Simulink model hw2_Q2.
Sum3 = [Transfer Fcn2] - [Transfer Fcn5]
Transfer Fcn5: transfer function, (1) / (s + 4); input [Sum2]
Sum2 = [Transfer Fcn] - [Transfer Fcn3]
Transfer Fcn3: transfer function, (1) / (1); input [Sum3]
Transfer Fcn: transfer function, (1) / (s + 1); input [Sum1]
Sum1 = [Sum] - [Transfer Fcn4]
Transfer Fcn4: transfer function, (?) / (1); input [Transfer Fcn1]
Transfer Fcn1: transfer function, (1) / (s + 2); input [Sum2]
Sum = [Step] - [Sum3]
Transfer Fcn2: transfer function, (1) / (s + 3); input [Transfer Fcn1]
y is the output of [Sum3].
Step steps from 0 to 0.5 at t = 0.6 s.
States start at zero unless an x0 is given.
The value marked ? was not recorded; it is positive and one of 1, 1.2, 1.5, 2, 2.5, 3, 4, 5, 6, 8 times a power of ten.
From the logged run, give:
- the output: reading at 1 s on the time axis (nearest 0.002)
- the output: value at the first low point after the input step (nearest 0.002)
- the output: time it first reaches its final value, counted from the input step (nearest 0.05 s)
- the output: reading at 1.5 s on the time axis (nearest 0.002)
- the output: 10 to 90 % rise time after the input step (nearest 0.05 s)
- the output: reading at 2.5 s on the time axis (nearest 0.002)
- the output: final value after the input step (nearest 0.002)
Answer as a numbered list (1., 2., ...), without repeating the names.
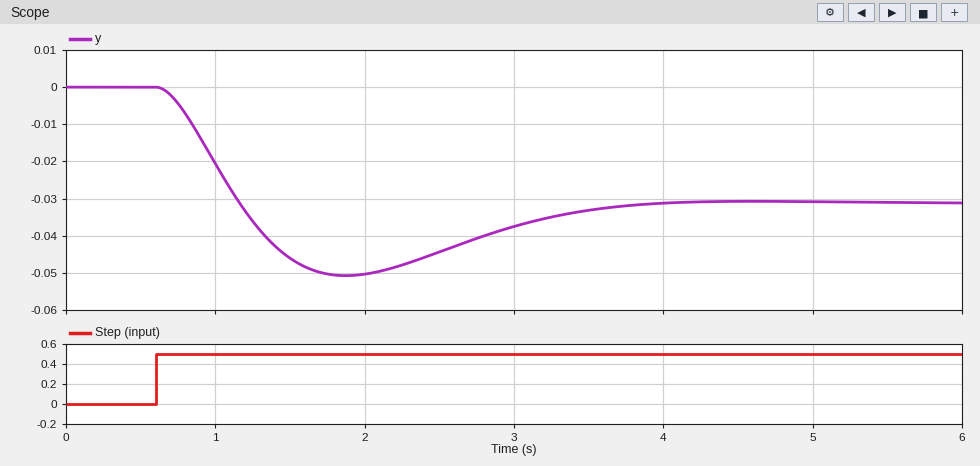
1. -0.020
2. -0.050
3. 0.55 s
4. -0.046
5. 0.40 s
6. -0.044
7. -0.032
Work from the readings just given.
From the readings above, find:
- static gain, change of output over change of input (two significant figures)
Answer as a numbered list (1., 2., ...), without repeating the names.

1. -0.064
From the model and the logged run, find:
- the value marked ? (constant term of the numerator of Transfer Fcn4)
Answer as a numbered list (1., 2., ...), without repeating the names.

1. 1
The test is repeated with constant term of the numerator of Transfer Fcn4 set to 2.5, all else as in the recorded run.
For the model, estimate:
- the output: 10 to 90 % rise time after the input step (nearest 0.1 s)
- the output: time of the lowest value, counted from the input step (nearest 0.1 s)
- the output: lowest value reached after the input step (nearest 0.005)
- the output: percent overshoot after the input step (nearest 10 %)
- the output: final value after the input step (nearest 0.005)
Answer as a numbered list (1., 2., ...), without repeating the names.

1. 0.3 s
2. 1.0 s
3. -0.040
4. 110 %
5. -0.020
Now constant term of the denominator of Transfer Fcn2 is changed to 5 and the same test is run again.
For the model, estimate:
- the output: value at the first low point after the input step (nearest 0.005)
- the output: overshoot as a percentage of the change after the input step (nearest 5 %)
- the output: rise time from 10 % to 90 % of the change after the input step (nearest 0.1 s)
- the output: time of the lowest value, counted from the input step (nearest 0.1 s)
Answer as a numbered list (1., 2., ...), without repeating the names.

1. -0.070
2. 10 %
3. 0.8 s
4. 1.9 s
